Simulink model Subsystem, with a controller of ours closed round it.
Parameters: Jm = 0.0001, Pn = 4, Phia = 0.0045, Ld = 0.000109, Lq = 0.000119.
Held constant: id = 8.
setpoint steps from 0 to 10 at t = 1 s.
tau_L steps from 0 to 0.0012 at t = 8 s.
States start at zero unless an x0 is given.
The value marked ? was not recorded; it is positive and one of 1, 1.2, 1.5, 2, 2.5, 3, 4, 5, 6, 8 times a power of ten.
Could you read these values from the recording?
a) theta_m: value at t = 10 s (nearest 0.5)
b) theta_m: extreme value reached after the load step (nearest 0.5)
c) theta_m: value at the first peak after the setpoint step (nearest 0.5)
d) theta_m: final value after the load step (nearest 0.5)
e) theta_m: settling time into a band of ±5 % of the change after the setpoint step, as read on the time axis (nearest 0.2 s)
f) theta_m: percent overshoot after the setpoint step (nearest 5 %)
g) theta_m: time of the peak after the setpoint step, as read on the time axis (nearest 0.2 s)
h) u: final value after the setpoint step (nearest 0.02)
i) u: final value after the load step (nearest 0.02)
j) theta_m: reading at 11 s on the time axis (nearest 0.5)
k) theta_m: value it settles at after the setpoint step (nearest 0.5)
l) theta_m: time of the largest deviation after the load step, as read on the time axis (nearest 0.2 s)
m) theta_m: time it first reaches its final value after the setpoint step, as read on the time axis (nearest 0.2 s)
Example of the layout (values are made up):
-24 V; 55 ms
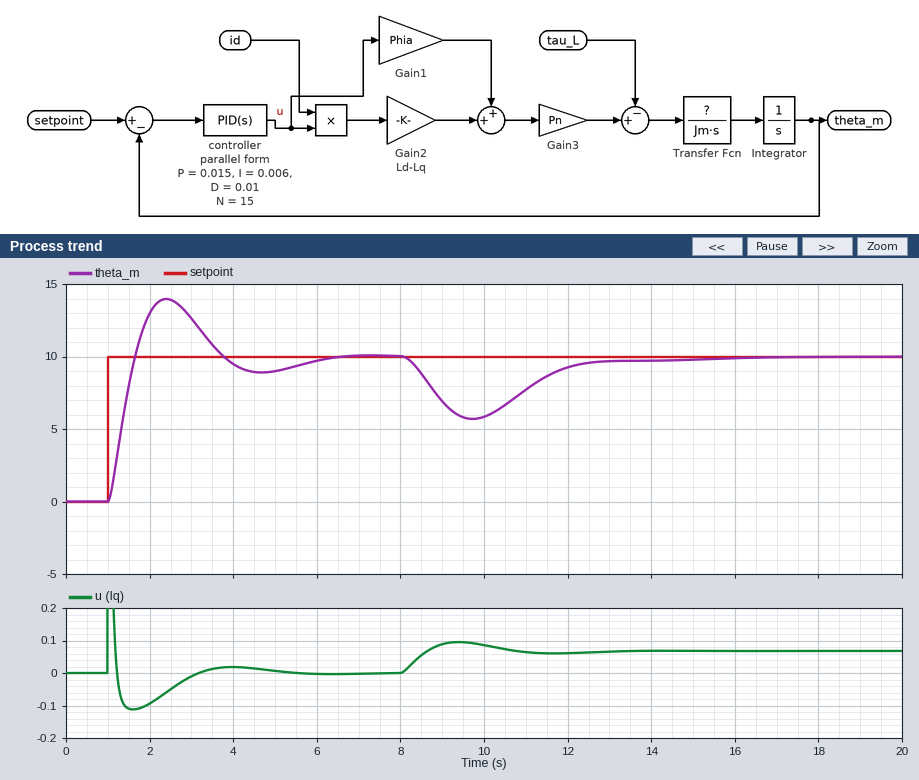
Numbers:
6.0; 5.5; 14.0; 10.0; 5.8 s; 40 %; 2.4 s; 0.00; 0.06; 7.5; 10.0; 9.8 s; 1.6 s
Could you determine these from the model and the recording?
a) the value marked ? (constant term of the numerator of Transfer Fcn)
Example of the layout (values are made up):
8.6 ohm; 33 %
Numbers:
1
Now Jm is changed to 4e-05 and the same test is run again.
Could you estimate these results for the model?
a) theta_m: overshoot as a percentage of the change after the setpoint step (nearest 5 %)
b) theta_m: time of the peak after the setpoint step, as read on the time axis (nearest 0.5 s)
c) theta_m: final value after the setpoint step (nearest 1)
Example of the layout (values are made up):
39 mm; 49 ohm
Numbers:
25 %; 1.5 s; 10
